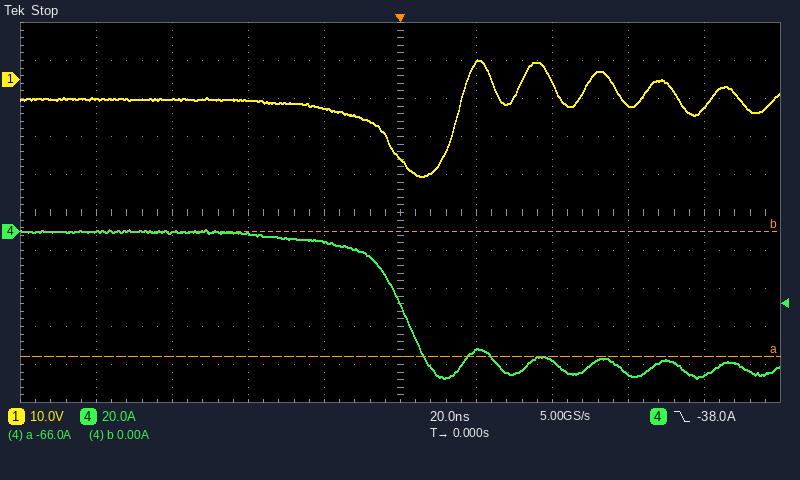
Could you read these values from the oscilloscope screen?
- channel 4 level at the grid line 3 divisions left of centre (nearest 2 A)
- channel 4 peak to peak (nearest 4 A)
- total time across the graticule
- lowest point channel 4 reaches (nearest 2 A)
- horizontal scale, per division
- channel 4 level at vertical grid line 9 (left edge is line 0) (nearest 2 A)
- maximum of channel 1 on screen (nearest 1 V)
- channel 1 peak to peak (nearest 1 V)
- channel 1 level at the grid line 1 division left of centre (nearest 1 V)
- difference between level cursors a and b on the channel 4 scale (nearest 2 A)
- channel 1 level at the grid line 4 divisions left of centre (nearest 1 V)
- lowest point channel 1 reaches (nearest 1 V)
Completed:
0 A
80 A
200 ns
-78 A
20 ns
-76 A
5 V
31 V
-8 V
66 A
-5 V
-26 V
